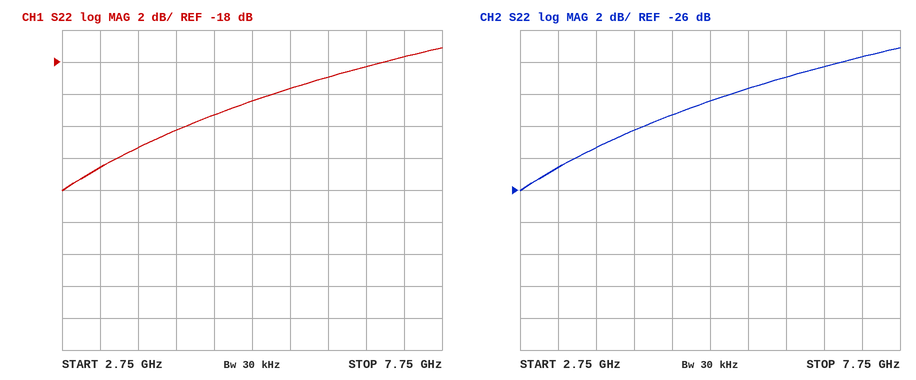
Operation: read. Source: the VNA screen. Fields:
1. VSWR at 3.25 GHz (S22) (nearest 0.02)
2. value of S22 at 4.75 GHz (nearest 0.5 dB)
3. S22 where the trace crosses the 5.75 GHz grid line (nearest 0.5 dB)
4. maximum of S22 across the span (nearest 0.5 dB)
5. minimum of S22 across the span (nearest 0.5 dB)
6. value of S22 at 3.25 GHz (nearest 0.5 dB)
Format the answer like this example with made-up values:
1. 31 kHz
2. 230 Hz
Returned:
1. 1.12
2. -21.5 dB
3. -19.5 dB
4. -17.0 dB
5. -26.0 dB
6. -24.5 dB
